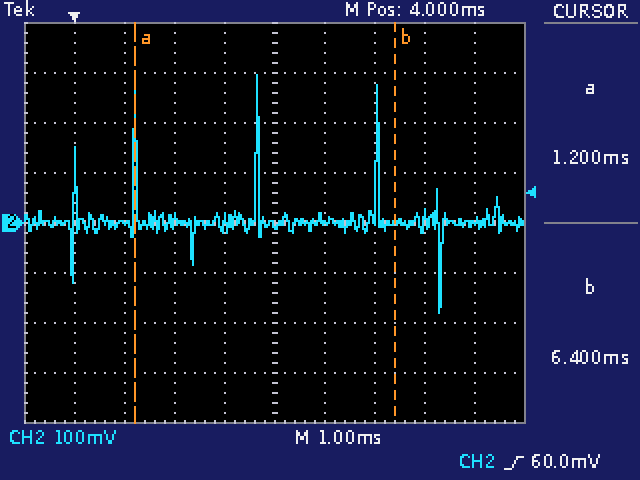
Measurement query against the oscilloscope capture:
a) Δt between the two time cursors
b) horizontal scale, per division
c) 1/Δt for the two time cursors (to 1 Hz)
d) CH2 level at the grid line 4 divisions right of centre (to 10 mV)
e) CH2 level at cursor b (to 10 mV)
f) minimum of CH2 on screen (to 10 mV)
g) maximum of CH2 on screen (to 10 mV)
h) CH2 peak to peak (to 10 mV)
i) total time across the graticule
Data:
5.2 ms
1 ms
192 Hz
0 mV
0 mV
-180 mV
300 mV
480 mV
10 ms
